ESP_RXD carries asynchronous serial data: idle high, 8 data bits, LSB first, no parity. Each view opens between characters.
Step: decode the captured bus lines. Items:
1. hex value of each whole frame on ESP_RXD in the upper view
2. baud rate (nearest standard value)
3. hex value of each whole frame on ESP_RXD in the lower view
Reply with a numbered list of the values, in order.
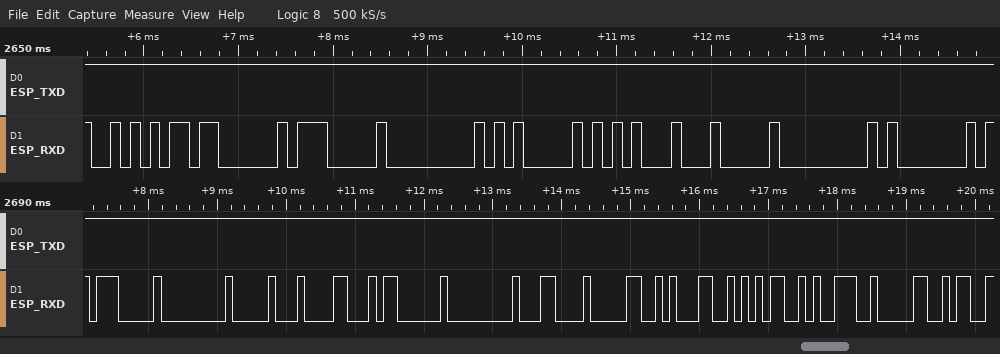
1. AA, 03, 07, 00, 05, 15, 04, 00, 01
2. 9600 baud
3. 07, 00, 10, 18, 03, 00, 0C, 30, 31, 35, 39, 30
